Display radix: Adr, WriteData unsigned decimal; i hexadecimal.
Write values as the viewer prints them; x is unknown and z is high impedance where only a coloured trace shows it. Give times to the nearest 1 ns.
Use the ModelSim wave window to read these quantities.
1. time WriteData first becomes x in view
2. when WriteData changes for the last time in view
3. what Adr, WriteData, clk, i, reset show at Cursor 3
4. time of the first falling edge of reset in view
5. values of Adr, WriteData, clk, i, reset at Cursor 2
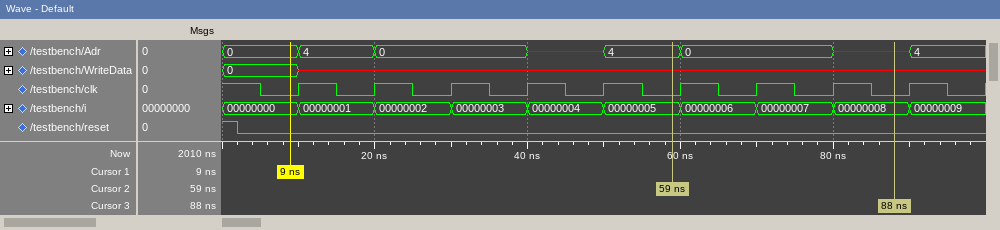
10 ns
10 ns
Adr=x, WriteData=x, clk=0, i=00000008, reset=0
2 ns
Adr=4, WriteData=x, clk=0, i=00000005, reset=0
